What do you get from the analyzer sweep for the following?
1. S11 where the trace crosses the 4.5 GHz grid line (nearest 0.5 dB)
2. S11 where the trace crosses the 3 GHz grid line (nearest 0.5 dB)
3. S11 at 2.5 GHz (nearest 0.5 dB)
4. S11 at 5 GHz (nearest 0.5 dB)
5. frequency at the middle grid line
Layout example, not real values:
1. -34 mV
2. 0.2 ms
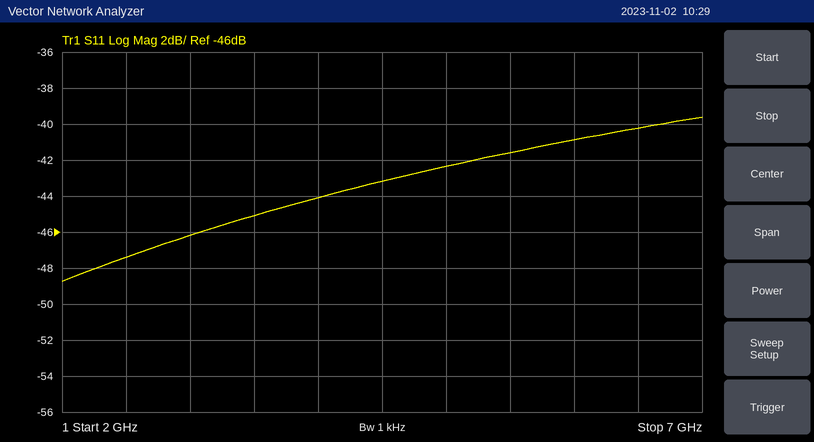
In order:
1. -43.0 dB
2. -46.0 dB
3. -47.5 dB
4. -42.5 dB
5. 4.5 GHz
